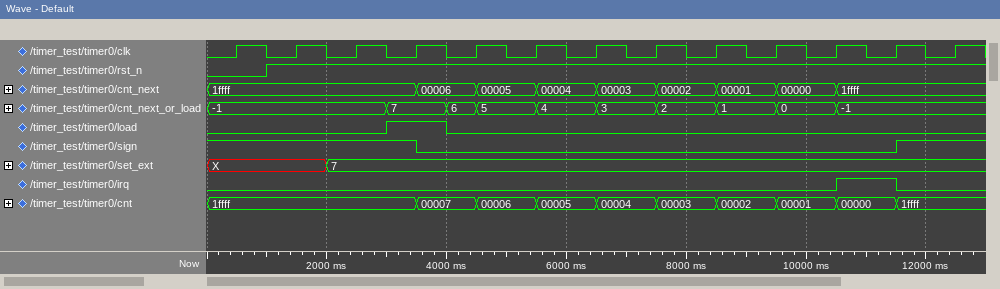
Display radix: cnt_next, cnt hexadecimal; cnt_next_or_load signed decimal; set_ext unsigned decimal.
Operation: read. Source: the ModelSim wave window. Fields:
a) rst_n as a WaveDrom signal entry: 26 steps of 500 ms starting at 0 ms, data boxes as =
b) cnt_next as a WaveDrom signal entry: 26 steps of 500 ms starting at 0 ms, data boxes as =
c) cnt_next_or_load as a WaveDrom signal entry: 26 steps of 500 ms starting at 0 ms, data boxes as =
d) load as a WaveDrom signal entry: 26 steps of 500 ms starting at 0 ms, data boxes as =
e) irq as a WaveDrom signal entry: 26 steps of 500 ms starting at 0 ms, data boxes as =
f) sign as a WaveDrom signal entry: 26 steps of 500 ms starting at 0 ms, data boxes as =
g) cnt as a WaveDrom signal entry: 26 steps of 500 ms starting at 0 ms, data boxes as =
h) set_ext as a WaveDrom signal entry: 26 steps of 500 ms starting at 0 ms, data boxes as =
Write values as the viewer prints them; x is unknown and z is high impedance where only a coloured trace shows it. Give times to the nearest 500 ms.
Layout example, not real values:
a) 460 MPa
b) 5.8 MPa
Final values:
a) {name: 'rst_n', wave: '0.1.......................'}
b) {name: 'cnt_next', wave: '=......=.=.=.=.=.=.=.=....', data: '1ffff 00006 00005 00004 00003 00002 00001 00000 1ffff'}
c) {name: 'cnt_next_or_load', wave: '=.....=.==.=.=.=.=.=.=....', data: '-1 7 6 5 4 3 2 1 0 -1'}
d) {name: 'load', wave: '0.....1.0.................'}
e) {name: 'irq', wave: '0....................1.0..'}
f) {name: 'sign', wave: '1......0...............1..'}
g) {name: 'cnt', wave: '=......=.=.=.=.=.=.=.=.=..', data: '1ffff 00007 00006 00005 00004 00003 00002 00001 00000 1ffff'}
h) {name: 'set_ext', wave: '=...=.....................', data: 'X 7'}
